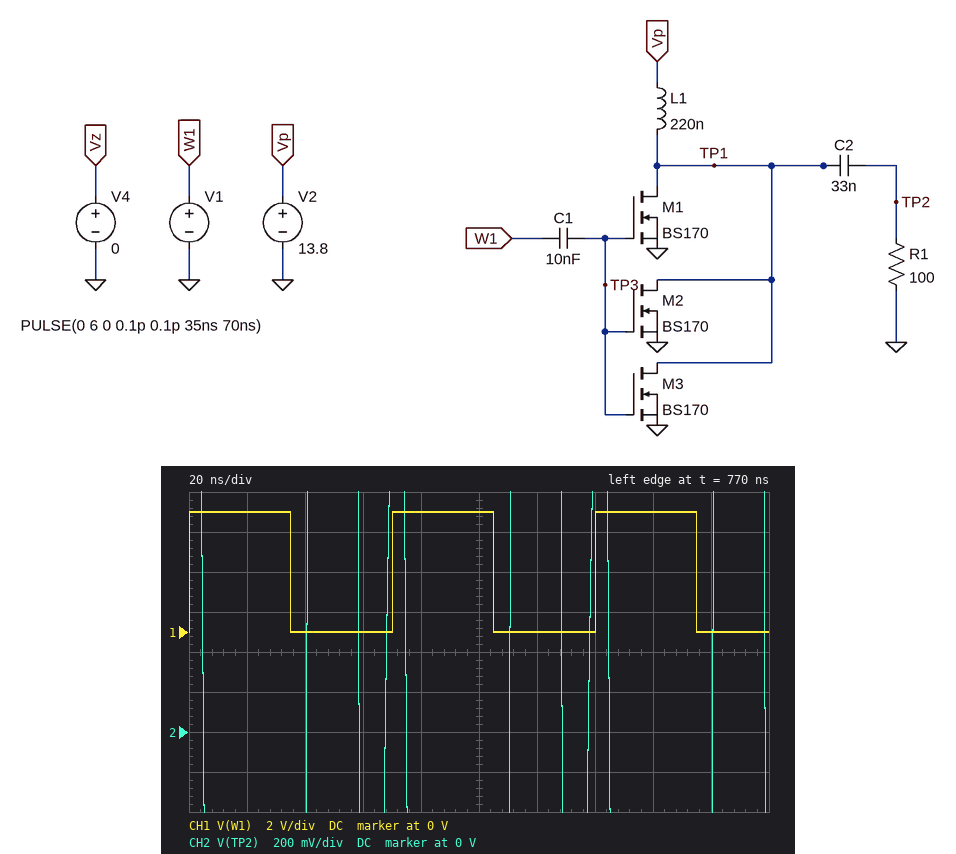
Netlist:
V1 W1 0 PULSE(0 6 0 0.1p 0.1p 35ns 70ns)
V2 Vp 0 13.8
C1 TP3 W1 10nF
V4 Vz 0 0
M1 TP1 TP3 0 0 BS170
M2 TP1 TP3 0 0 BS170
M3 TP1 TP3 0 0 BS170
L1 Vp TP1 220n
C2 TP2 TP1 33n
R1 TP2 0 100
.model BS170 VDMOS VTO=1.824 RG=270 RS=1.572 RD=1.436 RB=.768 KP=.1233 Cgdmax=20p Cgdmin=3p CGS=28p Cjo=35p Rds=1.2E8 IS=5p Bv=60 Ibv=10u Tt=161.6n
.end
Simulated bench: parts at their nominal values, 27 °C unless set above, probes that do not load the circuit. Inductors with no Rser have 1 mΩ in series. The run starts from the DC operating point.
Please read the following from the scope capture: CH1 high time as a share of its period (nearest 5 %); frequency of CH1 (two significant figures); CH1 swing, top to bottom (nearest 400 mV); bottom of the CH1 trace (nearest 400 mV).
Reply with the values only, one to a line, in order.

50 %
14 MHz
6.0 V
0 V
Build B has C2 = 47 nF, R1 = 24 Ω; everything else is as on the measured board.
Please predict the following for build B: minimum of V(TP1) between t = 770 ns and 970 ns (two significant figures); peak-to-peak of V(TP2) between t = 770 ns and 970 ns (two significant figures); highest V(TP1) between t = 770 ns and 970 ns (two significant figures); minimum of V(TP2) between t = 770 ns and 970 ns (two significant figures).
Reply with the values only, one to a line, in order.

3.6 V
29 V
32 V
-10 V
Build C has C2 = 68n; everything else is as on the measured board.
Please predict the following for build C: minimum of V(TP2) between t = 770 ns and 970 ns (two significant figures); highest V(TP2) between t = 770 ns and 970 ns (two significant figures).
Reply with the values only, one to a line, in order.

-8.8 V
37 V
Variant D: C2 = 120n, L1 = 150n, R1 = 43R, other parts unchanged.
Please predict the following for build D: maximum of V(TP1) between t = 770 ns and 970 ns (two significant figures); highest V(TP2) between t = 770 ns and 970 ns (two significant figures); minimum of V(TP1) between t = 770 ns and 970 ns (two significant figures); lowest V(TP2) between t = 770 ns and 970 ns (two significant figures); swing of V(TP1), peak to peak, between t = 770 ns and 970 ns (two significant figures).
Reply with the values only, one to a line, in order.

40 V
28 V
3.9 V
-8.3 V
36 V
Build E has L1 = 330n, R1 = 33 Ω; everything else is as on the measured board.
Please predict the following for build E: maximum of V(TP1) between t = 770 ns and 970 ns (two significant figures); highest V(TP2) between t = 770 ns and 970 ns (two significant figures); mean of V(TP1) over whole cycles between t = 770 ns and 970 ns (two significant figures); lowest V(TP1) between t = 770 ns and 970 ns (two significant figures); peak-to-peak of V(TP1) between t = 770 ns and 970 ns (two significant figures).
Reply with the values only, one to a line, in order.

34 V
21 V
14 V
2.4 V
32 V
